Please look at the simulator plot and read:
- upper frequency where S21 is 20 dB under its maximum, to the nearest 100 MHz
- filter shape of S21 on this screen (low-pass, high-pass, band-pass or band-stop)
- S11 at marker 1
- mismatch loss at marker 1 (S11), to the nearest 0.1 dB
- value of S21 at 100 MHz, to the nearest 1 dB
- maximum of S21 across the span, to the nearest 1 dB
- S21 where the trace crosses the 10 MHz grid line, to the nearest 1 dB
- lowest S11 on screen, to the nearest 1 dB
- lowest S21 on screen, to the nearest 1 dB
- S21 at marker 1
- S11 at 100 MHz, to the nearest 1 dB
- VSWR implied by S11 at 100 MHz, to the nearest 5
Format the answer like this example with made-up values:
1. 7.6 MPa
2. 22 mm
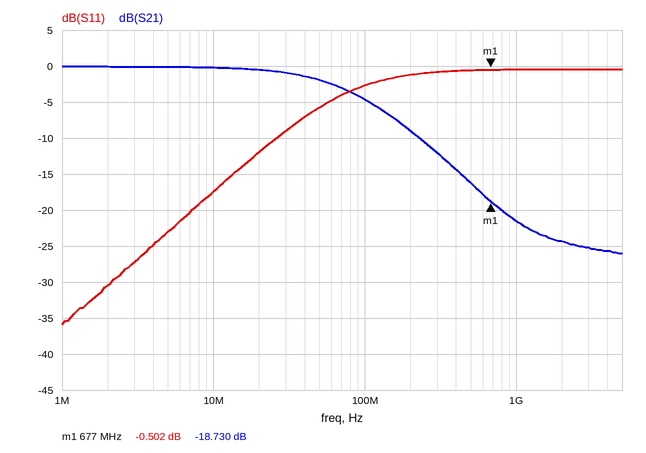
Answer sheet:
1. 800 MHz
2. low-pass
3. -0.502 dB
4. 9.6 dB
5. -5 dB
6. 0 dB
7. 0 dB
8. -36 dB
9. -26 dB
10. -18.730 dB
11. -3 dB
12. 5
